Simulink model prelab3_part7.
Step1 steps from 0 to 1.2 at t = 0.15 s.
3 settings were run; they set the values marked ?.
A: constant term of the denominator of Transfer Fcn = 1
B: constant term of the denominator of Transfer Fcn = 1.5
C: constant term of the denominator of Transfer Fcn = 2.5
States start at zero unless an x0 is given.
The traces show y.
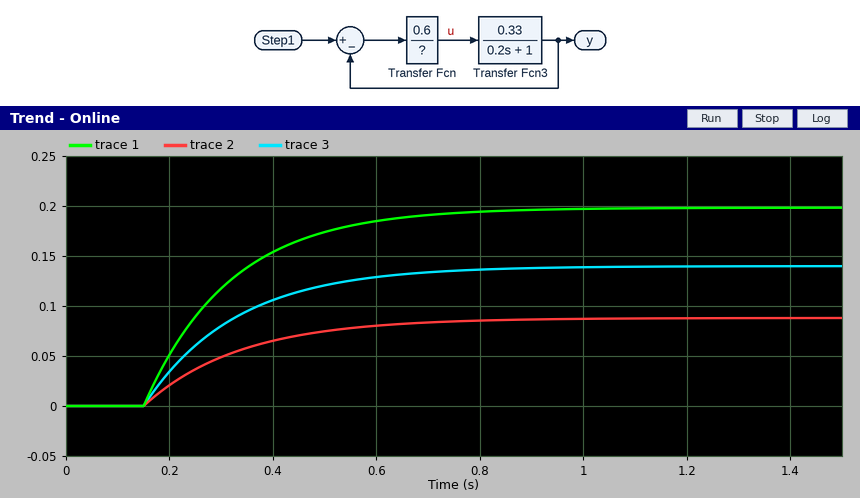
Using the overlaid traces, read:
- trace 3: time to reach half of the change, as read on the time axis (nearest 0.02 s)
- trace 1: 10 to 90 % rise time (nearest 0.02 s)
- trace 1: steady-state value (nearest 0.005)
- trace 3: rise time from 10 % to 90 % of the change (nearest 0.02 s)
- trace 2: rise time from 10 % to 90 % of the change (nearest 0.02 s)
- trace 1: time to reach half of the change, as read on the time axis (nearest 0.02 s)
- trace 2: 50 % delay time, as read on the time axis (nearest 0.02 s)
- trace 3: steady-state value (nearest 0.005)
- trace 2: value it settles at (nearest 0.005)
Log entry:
0.28 s
0.36 s
0.200
0.38 s
0.40 s
0.26 s
0.28 s
0.140
0.090
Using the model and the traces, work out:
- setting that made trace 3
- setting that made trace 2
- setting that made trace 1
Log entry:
B
C
A
